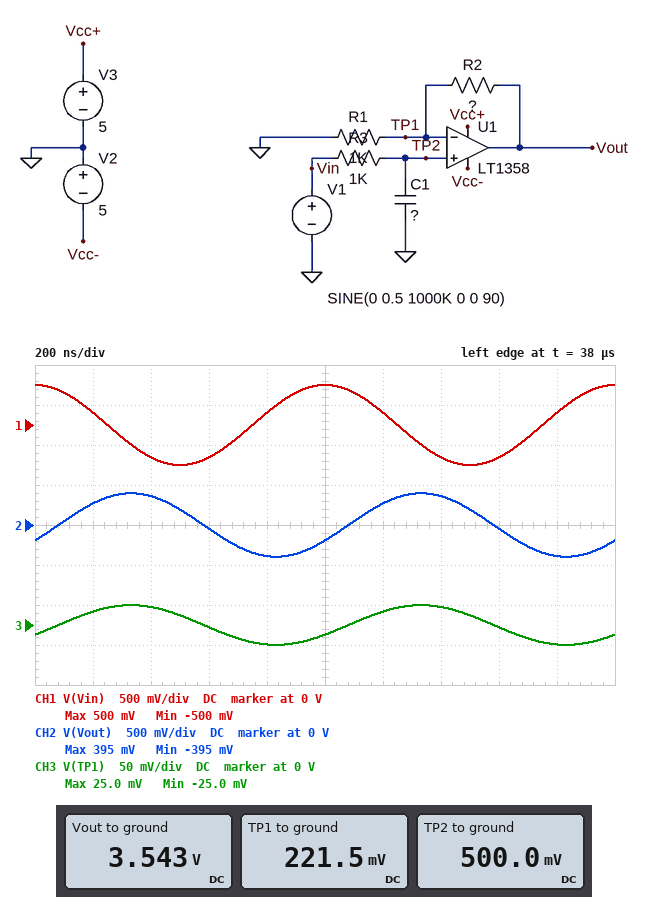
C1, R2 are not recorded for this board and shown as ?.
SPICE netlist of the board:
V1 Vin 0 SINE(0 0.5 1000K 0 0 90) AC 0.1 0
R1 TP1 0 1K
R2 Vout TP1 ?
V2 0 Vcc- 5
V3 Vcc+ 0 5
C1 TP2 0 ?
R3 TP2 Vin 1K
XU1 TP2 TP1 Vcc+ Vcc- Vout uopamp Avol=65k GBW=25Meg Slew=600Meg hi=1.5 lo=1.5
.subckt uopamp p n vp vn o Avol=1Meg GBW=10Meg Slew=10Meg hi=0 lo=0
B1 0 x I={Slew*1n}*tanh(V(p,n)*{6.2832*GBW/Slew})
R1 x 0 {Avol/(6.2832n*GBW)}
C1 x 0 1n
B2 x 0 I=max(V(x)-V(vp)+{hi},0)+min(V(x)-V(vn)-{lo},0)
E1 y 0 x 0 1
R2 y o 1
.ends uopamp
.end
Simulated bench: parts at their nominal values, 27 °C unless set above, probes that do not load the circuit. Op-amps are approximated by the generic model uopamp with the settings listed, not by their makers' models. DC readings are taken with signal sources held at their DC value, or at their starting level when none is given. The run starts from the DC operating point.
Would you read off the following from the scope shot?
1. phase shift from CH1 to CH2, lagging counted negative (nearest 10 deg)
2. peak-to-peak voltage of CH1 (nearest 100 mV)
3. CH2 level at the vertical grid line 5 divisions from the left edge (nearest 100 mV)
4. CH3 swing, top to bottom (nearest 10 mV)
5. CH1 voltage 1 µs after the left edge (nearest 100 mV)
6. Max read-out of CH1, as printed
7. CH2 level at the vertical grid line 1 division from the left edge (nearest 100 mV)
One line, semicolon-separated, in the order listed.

-120 deg; 1.0 V; -200 mV; 50 mV; 500 mV; 500 mV; 300 mV
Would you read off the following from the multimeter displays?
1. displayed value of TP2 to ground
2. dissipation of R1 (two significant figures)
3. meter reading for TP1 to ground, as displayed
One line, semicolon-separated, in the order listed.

500.0 mV; 49 µW; 221.5 mV
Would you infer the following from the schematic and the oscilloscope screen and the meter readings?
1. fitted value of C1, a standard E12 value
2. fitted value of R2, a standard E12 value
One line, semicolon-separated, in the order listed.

2.7 nF; 15 kΩ
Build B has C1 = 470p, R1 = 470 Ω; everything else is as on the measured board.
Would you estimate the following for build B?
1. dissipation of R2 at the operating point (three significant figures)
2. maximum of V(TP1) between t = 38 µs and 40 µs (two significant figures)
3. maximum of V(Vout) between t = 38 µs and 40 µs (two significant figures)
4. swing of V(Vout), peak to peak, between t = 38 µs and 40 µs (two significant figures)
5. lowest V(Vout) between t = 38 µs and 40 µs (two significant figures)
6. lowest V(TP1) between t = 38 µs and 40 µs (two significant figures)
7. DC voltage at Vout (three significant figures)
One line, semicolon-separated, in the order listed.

795 µW; 97 mV; 3.2 V; 6.4 V; -3.2 V; -97 mV; 3.56 V
